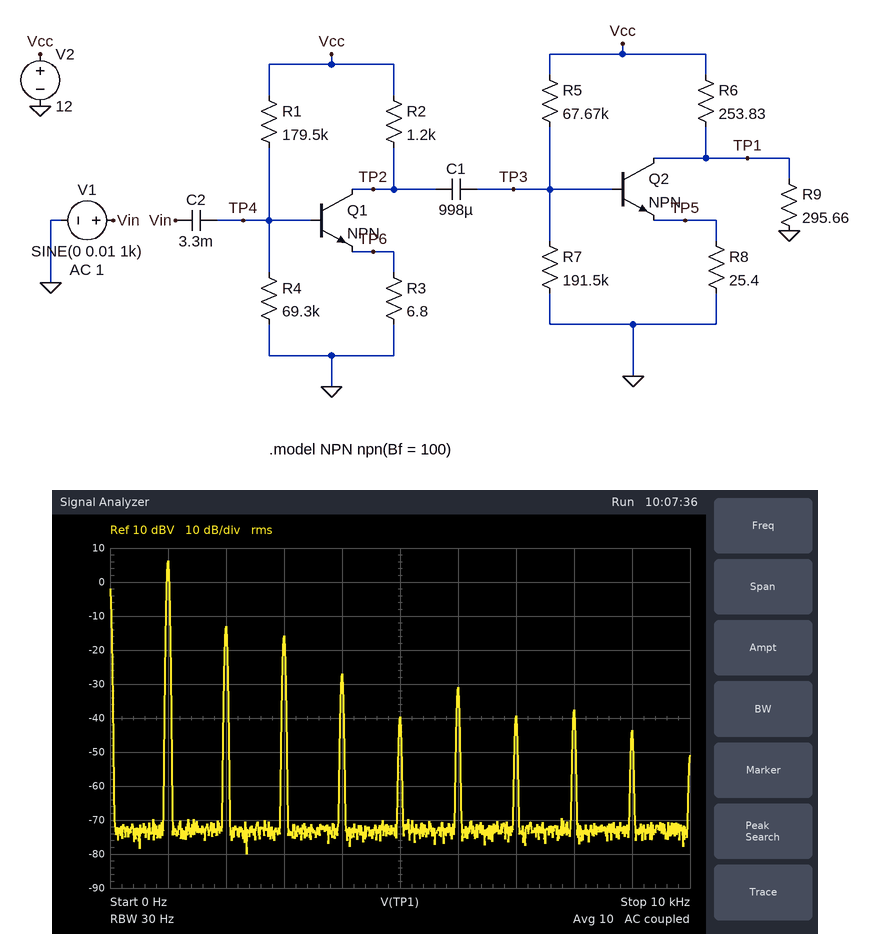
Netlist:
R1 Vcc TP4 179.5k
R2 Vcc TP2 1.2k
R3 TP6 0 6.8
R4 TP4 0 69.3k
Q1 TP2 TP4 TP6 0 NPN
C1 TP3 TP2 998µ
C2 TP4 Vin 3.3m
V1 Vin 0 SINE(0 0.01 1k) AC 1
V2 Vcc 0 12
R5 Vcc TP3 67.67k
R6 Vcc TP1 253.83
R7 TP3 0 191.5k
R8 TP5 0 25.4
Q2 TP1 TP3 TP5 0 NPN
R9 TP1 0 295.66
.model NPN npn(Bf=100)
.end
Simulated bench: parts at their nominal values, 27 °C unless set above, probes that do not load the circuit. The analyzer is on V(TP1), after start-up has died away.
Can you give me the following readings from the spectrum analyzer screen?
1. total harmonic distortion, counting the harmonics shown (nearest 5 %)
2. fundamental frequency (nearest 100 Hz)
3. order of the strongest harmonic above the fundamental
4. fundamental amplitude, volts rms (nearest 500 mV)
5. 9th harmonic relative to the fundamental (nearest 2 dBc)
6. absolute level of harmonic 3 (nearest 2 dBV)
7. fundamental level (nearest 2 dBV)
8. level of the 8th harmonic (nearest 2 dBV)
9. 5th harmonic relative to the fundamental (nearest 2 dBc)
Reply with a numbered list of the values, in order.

1. 15 %
2. 1.0 kHz
3. 2
4. 2.0 V
5. -50 dBc
6. -16 dBV
7. 6 dBV
8. -38 dBV
9. -46 dBc
